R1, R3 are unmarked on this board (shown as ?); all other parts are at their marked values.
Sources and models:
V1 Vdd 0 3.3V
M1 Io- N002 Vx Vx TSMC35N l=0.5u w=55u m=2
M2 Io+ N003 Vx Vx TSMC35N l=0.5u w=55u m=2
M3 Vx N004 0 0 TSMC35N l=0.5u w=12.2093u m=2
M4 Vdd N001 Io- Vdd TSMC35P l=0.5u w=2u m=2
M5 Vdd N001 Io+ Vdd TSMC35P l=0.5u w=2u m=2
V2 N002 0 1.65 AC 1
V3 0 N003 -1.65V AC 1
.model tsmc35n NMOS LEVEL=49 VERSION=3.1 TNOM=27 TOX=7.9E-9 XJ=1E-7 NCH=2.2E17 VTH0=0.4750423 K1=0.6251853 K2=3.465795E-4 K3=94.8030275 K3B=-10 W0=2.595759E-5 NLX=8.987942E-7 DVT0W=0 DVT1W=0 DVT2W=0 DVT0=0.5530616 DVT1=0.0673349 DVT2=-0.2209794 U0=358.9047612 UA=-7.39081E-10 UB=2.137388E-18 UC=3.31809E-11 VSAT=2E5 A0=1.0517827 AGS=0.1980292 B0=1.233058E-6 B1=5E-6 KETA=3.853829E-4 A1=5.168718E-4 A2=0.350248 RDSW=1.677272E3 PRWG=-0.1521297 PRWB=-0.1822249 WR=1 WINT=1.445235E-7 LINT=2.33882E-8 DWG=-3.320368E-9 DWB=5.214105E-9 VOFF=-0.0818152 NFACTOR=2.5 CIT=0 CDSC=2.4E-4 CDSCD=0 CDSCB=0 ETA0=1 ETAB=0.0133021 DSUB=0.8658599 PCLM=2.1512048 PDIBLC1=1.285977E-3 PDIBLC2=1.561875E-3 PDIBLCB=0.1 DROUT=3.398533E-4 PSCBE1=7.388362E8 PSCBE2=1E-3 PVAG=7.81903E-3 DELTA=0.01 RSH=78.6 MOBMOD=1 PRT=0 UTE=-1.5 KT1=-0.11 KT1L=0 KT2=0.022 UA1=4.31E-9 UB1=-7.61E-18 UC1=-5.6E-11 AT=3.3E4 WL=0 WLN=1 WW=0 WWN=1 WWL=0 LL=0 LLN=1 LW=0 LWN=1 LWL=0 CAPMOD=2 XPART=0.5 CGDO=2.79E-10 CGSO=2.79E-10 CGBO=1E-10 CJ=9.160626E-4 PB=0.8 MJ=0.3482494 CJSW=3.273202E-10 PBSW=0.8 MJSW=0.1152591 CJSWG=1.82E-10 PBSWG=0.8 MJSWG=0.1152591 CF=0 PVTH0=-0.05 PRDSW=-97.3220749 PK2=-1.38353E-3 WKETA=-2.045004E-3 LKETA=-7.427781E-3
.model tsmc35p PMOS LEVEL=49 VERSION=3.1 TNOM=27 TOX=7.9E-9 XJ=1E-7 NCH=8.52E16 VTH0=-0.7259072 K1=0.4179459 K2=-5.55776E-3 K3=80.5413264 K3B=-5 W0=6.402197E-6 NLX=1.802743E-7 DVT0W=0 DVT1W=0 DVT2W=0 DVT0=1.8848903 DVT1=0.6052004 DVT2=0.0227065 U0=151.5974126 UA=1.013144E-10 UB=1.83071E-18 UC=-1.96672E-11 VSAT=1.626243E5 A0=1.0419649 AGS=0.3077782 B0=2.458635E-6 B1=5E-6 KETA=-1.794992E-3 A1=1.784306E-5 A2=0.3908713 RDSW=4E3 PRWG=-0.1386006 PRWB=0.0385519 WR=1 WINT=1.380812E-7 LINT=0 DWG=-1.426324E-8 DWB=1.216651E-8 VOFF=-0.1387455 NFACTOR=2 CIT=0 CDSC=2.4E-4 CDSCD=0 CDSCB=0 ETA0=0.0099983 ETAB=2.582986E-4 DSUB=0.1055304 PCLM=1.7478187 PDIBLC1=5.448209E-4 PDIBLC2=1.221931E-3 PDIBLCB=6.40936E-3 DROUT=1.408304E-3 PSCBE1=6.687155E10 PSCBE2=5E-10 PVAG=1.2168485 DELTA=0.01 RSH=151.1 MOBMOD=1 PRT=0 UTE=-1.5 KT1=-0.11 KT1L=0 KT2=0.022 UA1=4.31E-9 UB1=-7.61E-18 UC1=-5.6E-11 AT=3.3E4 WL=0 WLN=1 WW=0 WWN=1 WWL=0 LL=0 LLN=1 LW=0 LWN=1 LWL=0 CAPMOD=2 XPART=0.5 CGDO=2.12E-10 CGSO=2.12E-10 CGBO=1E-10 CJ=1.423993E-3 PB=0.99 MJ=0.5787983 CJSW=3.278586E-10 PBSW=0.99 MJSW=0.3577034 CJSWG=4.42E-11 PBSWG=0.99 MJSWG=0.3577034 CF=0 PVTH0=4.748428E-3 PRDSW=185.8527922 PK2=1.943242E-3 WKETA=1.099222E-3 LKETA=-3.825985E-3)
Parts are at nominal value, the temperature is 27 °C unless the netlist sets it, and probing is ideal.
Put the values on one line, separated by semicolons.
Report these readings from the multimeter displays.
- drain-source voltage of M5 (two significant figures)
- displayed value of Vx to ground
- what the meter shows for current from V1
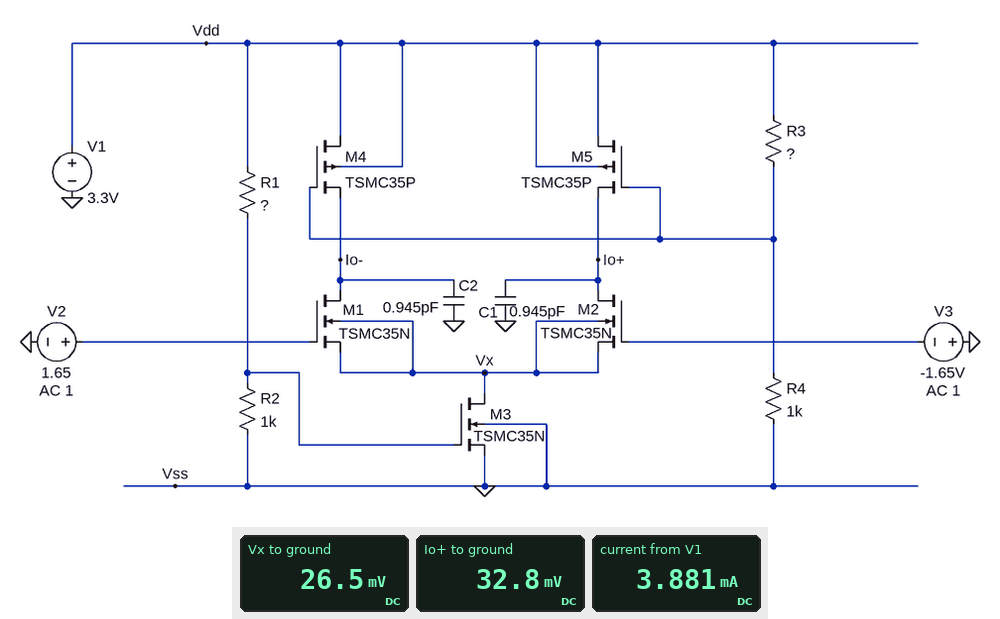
3.3 V; 26.5 mV; 3.881 mA
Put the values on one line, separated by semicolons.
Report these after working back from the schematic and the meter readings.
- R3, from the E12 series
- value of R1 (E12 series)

680 Ω; 820 Ω
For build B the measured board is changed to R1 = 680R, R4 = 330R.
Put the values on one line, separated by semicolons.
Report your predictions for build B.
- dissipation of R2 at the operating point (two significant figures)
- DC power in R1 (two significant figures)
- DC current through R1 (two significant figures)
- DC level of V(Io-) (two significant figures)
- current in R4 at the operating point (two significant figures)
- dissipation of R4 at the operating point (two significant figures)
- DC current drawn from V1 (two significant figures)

3.9 mW; 2.6 mW; 2.0 mA; 150 mV; 3.3 mA; 3.5 mW; 5.7 mA
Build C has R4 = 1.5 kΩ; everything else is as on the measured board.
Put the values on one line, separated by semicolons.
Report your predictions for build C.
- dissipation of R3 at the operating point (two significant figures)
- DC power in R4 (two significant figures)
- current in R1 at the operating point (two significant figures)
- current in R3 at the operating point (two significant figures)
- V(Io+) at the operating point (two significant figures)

1.6 mW; 3.4 mW; 1.8 mA; 1.5 mA; 8.3 mV
